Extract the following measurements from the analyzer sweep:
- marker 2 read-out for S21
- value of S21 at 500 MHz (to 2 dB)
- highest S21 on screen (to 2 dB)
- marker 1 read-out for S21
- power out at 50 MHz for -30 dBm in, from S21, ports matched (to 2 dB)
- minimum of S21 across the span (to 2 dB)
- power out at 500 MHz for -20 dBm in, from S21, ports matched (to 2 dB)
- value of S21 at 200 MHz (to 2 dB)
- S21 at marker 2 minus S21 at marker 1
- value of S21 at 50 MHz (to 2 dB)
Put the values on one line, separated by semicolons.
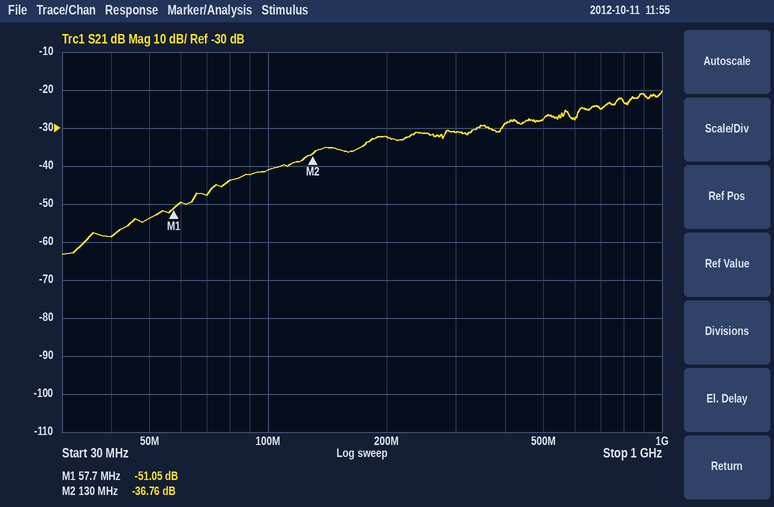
-36.76 dB; -28 dB; -20 dB; -51.05 dB; -84 dBm; -64 dB; -48 dBm; -32 dB; 14.29 dB; -54 dB
